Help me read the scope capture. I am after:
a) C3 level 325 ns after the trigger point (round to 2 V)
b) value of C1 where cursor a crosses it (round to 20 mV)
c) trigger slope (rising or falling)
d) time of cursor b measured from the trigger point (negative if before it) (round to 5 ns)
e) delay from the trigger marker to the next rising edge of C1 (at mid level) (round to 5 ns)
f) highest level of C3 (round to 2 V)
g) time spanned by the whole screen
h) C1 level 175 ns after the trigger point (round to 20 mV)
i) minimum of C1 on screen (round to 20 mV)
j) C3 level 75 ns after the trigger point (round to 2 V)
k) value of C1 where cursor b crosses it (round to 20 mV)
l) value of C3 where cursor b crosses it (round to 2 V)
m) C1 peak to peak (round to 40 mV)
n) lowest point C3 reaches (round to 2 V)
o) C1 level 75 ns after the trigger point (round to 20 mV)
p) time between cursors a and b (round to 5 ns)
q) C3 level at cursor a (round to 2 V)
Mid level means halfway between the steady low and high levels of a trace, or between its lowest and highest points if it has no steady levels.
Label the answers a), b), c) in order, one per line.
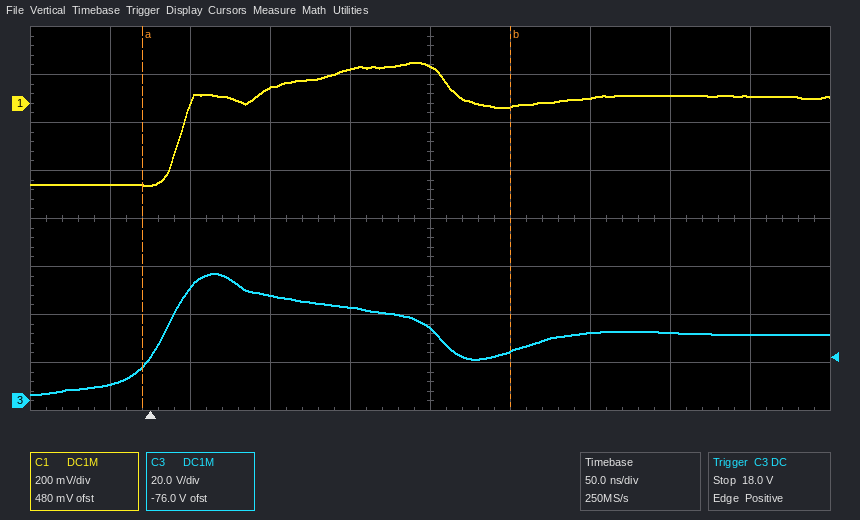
a) 28 V
b) -340 mV
c) rising
d) +225 ns
e) 20 ns
f) 54 V
g) 500 ns
h) 160 mV
i) -340 mV
j) 44 V
k) -20 mV
l) 20 V
m) 520 mV
n) 2 V
o) 60 mV
p) 230 ns
q) 14 V
